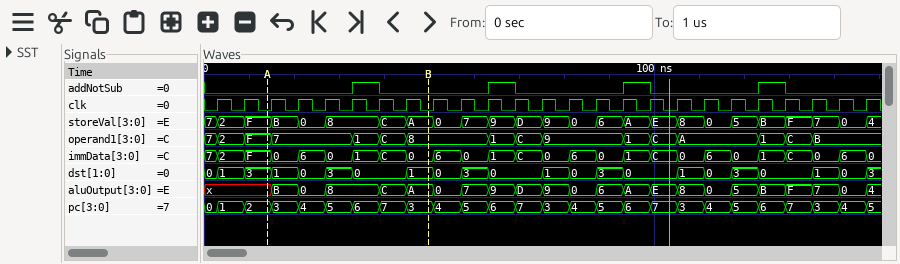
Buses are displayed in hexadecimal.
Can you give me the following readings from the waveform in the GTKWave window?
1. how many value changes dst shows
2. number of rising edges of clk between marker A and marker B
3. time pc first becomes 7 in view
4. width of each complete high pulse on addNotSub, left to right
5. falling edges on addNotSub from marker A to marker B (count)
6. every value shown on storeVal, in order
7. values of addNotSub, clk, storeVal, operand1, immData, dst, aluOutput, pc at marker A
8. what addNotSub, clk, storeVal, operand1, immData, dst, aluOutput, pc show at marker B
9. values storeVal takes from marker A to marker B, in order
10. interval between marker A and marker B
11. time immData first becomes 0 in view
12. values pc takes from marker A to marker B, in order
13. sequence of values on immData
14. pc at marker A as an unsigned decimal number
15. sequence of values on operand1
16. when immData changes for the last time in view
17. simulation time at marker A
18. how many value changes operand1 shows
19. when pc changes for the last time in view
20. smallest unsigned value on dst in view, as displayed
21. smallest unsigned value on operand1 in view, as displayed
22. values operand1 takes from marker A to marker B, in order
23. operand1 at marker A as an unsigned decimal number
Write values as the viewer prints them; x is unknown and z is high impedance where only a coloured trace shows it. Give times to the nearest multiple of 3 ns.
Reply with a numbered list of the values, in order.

1. 21
2. 6
3. 39 ns
4. 6 ns, 6 ns, 6 ns, 6 ns
5. 1
6. 7, 2, F, B, 0, 8, C, A, 0, 7, 9, D, 9, 0, 6, A, E, 8, 0, 5, B, F, 7, 0, 4
7. addNotSub=0, clk=0, storeVal=F, operand1=F, immData=F, dst=3, aluOutput=x, pc=2
8. addNotSub=0, clk=0, storeVal=A, operand1=8, immData=0, dst=1, aluOutput=A, pc=3
9. F, B, 0, 8, C, A
10. 36 ns
11. 15 ns
12. 2, 3, 4, 5, 6, 7, 3
13. 7, 2, F, 0, 6, 0, 1, C, 0, 6, 0, 1, C, 0, 6, 0, 1, C, 0, 6, 0, 1, C, 0, 6, 0
14. 2
15. 7, 2, F, 7, 1, C, 8, 1, C, 9, 1, C, A, 1, C, B
16. 147 ns
17. 15 ns
18. 15
19. 147 ns
20. 0
21. 1
22. F, 7, 1, C, 8
23. 15
